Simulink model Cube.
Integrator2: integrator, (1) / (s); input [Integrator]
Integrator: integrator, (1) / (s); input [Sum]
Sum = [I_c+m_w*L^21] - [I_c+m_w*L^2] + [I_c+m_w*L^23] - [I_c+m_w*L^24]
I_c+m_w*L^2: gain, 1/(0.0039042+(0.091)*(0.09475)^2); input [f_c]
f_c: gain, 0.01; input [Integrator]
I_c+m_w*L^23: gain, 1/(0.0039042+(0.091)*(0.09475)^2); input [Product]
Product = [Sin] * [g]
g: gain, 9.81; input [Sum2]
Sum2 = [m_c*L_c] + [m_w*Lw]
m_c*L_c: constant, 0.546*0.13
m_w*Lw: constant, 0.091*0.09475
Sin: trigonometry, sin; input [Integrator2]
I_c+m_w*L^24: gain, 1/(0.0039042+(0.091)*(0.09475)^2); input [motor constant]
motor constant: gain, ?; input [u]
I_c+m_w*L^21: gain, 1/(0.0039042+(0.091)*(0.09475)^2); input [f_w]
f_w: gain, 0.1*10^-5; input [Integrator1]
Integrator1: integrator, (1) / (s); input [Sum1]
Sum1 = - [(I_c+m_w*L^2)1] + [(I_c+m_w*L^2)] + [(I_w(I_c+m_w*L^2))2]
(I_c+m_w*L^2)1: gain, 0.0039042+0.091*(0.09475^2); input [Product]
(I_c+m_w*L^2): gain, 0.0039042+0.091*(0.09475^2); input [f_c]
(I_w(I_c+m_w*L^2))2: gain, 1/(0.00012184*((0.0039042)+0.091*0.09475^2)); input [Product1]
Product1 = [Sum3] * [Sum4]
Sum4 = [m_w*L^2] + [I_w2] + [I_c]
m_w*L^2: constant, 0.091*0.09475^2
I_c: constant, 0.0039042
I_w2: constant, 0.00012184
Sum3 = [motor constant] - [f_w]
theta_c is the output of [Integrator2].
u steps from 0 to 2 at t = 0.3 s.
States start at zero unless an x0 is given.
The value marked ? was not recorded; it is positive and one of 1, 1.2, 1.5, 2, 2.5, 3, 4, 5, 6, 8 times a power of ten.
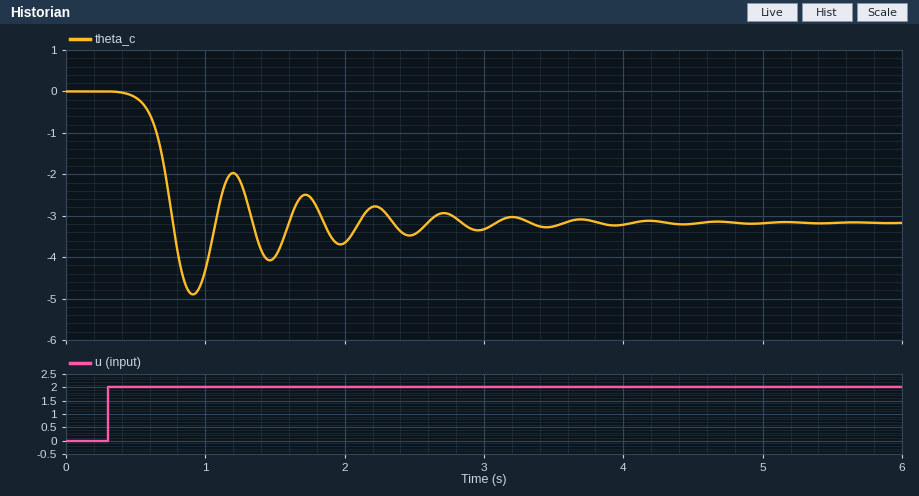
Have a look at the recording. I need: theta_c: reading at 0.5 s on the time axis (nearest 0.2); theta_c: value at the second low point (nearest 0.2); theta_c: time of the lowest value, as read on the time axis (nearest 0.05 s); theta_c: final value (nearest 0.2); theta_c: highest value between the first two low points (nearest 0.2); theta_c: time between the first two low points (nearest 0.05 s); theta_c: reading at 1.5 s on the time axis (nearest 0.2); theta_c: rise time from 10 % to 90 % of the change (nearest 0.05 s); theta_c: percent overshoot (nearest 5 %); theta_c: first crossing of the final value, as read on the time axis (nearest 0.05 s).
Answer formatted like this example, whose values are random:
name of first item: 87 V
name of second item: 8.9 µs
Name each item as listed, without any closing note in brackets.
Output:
theta_c: reading at 0.5 s on the time axis: -0.2
theta_c: value at the second low point: -4.0
theta_c: time of the lowest value, as read on the time axis: 0.90 s
theta_c: final value: -3.2
theta_c: highest value between the first two low points: -2.0
theta_c: time between the first two low points: 0.55 s
theta_c: reading at 1.5 s on the time axis: -4.0
theta_c: rise time from 10 % to 90 % of the change: 0.20 s
theta_c: percent overshoot: 55 %
theta_c: first crossing of the final value, as read on the time axis: 0.75 s
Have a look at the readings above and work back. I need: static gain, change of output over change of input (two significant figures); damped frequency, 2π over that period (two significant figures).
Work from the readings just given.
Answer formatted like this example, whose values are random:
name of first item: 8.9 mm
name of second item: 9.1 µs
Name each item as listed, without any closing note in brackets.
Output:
static gain, change of output over change of input: -1.6
damped frequency, 2π over that period: 11 rad/s
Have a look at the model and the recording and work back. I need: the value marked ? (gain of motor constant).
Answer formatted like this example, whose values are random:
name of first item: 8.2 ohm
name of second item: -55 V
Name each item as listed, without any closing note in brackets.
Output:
the value marked ?: 0.012
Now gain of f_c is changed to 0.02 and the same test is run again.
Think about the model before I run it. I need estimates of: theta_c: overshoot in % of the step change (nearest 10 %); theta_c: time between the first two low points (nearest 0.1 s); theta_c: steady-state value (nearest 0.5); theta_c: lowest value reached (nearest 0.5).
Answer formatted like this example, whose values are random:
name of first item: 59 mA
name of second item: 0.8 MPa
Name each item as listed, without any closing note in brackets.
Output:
theta_c: overshoot in % of the step change: 40 %
theta_c: time between the first two low points: 0.5 s
theta_c: steady-state value: -3.0
theta_c: lowest value reached: -4.5
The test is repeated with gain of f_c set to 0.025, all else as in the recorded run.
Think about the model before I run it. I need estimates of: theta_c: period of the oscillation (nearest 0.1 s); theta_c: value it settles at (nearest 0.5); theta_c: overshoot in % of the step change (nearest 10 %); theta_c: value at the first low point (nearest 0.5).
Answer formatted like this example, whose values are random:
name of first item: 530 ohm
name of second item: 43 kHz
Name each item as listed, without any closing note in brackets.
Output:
theta_c: period of the oscillation: 0.5 s
theta_c: value it settles at: -3.0
theta_c: overshoot in % of the step change: 30 %
theta_c: value at the first low point: -4.0
